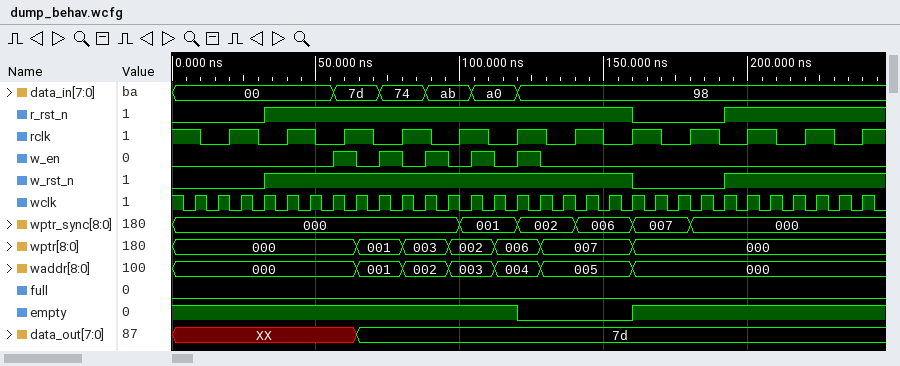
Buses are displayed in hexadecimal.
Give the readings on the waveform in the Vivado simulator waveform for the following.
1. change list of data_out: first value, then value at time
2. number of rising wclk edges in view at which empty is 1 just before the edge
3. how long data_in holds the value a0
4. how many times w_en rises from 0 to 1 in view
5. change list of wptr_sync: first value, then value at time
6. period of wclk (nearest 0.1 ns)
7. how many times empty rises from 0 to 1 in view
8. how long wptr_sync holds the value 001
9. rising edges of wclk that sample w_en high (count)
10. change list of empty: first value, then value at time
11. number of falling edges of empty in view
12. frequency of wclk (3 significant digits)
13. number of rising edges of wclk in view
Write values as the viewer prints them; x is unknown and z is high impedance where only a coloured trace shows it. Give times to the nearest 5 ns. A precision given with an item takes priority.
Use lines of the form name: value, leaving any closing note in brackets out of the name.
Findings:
change list of data_out: first value, then value at time: XX, 7d at 65 ns
number of rising wclk edges in view at which empty is 1 just before the edge: 25
how long data_in holds the value a0: 15 ns
how many times w_en rises from 0 to 1 in view: 5
change list of wptr_sync: first value, then value at time: 000, 001 at 100 ns, 002 at 120 ns, 006 at 140 ns, 007 at 160 ns, 000 at 180 ns
period of wclk: 8 ns
how many times empty rises from 0 to 1 in view: 1
how long wptr_sync holds the value 001: 20 ns
rising edges of wclk that sample w_en high: 5
change list of empty: first value, then value at time: 1, 0 at 120 ns, 1 at 160 ns
number of falling edges of empty in view: 1
frequency of wclk: 125 MHz
number of rising edges of wclk in view: 30
